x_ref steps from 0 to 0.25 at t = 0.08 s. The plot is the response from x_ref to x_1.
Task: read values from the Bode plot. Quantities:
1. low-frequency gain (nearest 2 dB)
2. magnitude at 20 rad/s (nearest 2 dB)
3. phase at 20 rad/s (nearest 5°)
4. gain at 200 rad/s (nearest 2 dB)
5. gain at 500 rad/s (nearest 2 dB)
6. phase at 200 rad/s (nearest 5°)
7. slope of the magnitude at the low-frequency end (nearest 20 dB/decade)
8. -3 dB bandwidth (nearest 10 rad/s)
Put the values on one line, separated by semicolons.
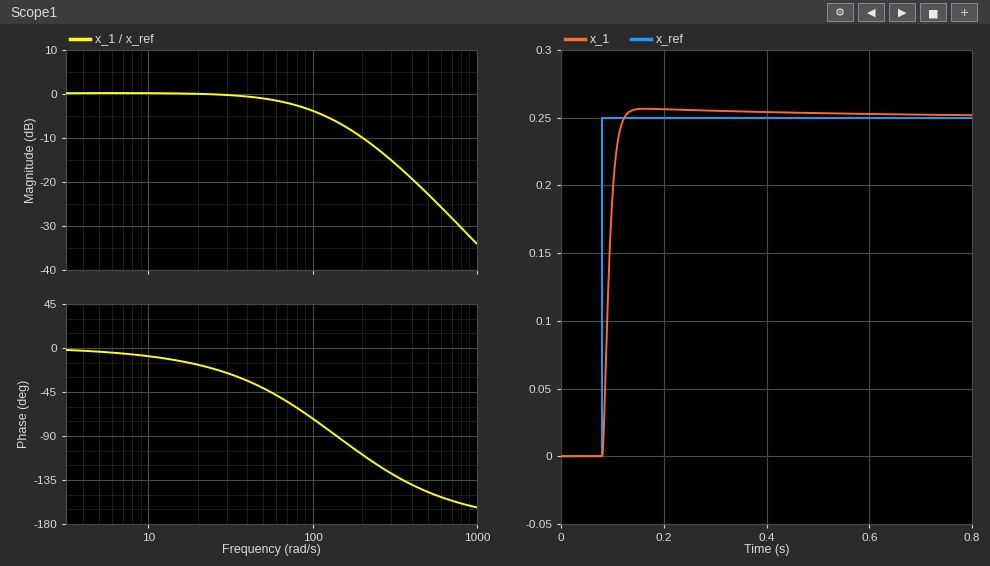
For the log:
0 dB; 0 dB; -15°; -10 dB; -22 dB; -110°; 0 dB/decade; 80 rad/s
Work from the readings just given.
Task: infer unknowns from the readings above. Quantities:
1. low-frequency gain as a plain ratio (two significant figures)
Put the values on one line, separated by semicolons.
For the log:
1.0
